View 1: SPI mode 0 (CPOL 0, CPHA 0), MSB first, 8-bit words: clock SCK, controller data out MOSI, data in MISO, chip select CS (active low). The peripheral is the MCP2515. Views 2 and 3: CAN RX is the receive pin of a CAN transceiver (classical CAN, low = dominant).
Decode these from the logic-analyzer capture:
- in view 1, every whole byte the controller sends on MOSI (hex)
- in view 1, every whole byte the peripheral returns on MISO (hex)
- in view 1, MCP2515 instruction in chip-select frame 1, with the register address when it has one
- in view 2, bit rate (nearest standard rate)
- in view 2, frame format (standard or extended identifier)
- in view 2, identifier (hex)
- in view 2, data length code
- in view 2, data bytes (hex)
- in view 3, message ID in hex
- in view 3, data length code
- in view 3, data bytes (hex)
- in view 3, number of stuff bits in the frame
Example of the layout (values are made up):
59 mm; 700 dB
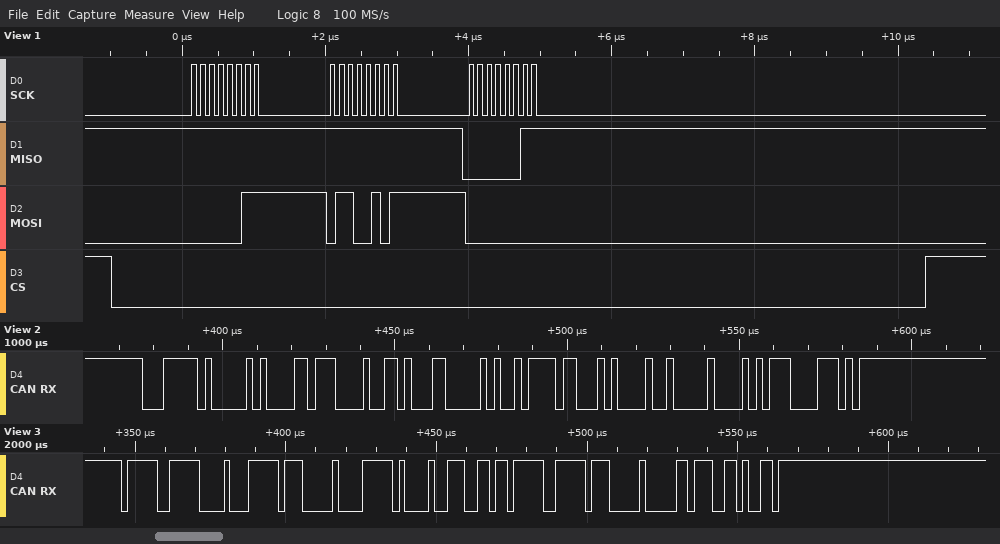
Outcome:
03 65 00; FF FF 03; READ 0x65; 500 kbit/s; standard; 0x1F8; 8; 6E 13 46 04 BD 8A 12 00; 0x7DF; 8; FF 00 7E 13 9B 7D FE 00; 9
